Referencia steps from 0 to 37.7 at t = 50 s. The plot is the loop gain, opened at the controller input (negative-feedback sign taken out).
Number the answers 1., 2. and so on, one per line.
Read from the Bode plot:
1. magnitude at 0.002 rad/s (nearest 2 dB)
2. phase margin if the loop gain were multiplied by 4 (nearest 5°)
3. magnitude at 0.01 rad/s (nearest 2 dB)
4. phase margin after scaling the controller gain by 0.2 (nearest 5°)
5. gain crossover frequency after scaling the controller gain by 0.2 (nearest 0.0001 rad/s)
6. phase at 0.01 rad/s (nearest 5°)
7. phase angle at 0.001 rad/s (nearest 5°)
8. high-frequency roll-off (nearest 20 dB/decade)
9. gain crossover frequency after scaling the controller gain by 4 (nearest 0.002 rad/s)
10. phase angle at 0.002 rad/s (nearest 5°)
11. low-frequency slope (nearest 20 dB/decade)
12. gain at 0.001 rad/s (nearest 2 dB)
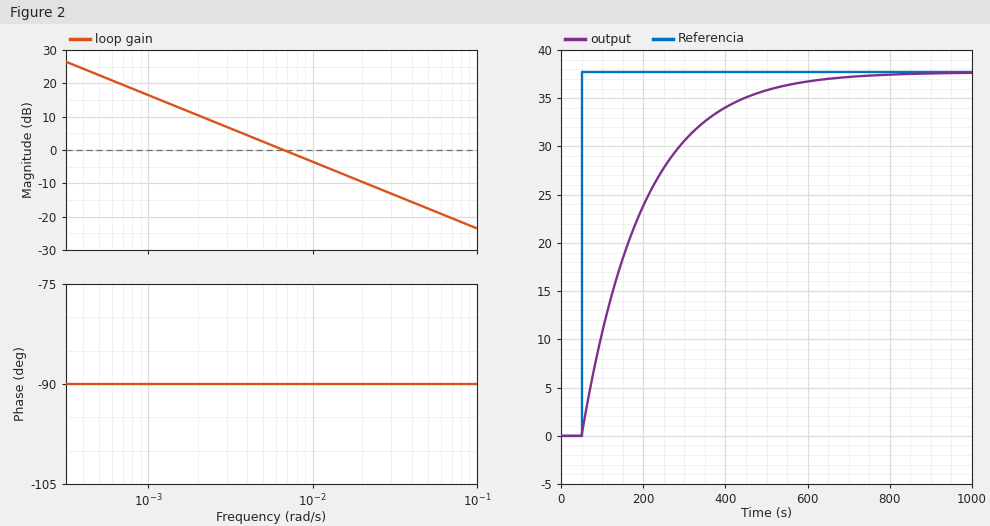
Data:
1. 10 dB
2. 90°
3. -4 dB
4. 90°
5. 0.0013 rad/s
6. -90°
7. -90°
8. -20 dB/decade
9. 0.026 rad/s
10. -90°
11. -20 dB/decade
12. 16 dB
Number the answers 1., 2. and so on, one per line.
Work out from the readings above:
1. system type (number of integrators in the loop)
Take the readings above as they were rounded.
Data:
1. 1
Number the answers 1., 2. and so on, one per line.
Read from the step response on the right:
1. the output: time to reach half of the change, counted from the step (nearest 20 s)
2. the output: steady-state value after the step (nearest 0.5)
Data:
1. 100 s
2. 37.5
